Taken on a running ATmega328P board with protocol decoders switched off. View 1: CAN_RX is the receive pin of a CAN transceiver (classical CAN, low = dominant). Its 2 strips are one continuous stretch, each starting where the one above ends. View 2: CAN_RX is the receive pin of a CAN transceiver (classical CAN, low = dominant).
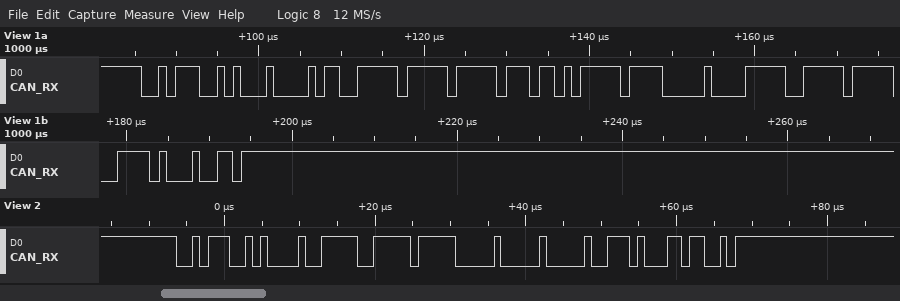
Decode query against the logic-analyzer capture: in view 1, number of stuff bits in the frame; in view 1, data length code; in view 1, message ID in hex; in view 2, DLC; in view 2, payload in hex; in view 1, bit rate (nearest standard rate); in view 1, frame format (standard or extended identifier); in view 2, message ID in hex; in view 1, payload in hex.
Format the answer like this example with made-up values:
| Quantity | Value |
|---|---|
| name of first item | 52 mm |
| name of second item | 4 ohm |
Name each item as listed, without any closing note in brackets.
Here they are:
| Quantity | Value |
|---|---|
| in view 1, number of stuff bits in the frame | 8 |
| in view 1, data length code | 8 |
| in view 1, message ID in hex | 0x2E5 |
| in view 2, DLC | 4 |
| in view 2, payload in hex | FB FF 00 00 |
| in view 1, bit rate | 1000 kbit/s |
| in view 1, frame format | standard |
| in view 2, message ID in hex | 0x2E5 |
| in view 1, payload in hex | 59 FF FF B5 FF 00 7D FF |
